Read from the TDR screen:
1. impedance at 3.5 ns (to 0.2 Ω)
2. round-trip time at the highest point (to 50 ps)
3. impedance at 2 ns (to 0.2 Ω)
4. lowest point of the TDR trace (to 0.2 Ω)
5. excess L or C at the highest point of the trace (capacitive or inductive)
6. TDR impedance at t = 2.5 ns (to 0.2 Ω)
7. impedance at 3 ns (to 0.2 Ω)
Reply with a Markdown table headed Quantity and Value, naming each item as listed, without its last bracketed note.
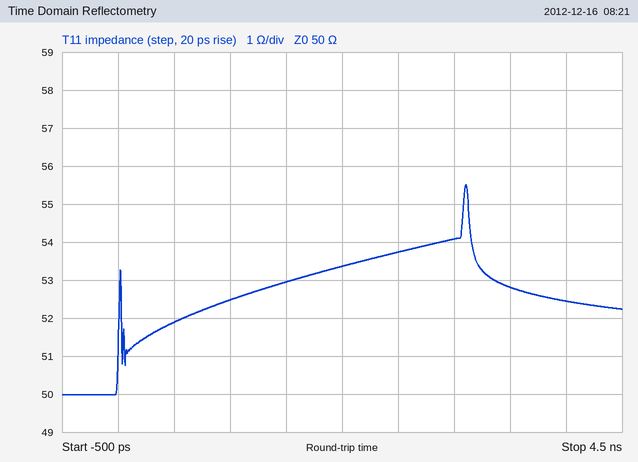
| Quantity | Value |
|---|---|
| impedance at 3.5 ns | 52.8 Ω |
| round-trip time at the highest point | 3.10 ns |
| impedance at 2 ns | 53.4 Ω |
| lowest point of the TDR trace | 50.0 Ω |
| excess L or C at the highest point of the trace | inductive |
| TDR impedance at t = 2.5 ns | 53.8 Ω |
| impedance at 3 ns | 54.0 Ω |
